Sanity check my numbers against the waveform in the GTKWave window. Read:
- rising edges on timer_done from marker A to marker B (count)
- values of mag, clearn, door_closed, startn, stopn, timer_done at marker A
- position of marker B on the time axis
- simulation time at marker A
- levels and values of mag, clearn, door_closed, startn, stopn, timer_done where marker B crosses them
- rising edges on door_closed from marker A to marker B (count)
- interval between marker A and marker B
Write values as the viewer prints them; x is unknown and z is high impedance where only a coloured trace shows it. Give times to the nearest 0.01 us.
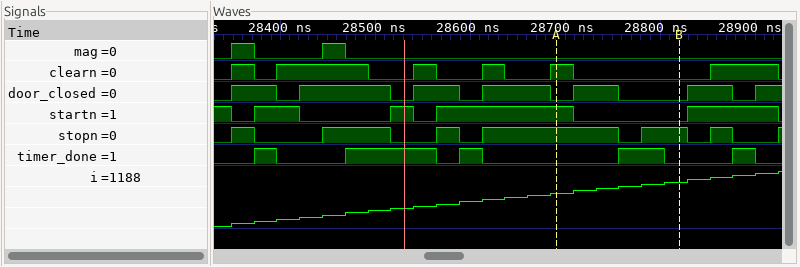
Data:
1
mag=0, clearn=1, door_closed=0, startn=1, stopn=1, timer_done=0
28.82 us
28.69 us
mag=0, clearn=0, door_closed=0, startn=0, stopn=1, timer_done=0
1
0.13 us
